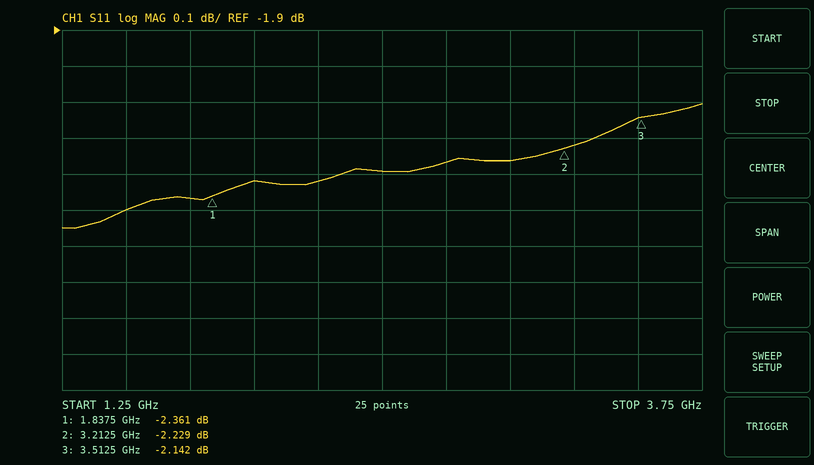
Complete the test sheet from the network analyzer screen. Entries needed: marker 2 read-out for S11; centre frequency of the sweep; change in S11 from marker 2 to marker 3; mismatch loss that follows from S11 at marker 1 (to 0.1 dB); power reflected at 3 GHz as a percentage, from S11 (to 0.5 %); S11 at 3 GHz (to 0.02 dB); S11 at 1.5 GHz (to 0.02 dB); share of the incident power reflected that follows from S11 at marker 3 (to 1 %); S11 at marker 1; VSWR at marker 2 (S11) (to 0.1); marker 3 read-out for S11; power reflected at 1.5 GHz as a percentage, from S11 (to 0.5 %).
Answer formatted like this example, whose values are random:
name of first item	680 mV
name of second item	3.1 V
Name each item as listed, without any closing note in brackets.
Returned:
marker 2 read-out for S11	-2.229 dB
centre frequency of the sweep	2.5 GHz
change in S11 from marker 2 to marker 3	0.087 dB
mismatch loss that follows from S11 at marker 1	3.8 dB
power reflected at 3 GHz as a percentage, from S11	59.5 %
S11 at 3 GHz	-2.26 dB
S11 at 1.5 GHz	-2.40 dB
share of the incident power reflected that follows from S11 at marker 3	61 %
S11 at marker 1	-2.361 dB
VSWR at marker 2 (S11)	7.8
marker 3 read-out for S11	-2.142 dB
power reflected at 1.5 GHz as a percentage, from S11	57.5 %
